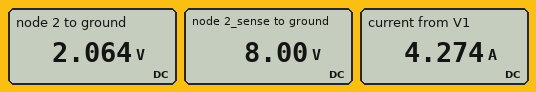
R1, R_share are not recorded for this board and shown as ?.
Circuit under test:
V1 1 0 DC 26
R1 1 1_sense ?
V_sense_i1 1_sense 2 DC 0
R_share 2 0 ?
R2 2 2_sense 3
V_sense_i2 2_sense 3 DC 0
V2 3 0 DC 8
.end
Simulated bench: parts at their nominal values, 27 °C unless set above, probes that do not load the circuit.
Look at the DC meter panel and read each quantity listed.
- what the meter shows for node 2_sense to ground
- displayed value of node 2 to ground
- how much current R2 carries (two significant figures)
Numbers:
8.00 V
2.064 V
2.0 A
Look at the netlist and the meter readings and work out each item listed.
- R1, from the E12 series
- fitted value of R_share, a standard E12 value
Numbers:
5.6 Ω
0.33 Ω
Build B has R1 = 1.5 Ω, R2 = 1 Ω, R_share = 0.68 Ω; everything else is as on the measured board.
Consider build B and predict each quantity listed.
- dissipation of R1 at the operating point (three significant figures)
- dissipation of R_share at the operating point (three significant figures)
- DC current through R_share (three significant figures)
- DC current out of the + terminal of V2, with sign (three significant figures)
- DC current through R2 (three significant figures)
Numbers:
214 W
95.9 W
11.9 A
-75.0 mA
75.0 mA
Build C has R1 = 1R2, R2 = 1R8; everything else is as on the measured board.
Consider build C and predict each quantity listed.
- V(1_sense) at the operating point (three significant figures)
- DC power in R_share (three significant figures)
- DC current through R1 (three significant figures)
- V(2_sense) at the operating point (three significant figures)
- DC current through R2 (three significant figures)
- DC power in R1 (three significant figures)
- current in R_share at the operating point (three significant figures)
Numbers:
5.91 V
106 W
16.7 A
8.00 V
1.16 A
336 W
17.9 A
